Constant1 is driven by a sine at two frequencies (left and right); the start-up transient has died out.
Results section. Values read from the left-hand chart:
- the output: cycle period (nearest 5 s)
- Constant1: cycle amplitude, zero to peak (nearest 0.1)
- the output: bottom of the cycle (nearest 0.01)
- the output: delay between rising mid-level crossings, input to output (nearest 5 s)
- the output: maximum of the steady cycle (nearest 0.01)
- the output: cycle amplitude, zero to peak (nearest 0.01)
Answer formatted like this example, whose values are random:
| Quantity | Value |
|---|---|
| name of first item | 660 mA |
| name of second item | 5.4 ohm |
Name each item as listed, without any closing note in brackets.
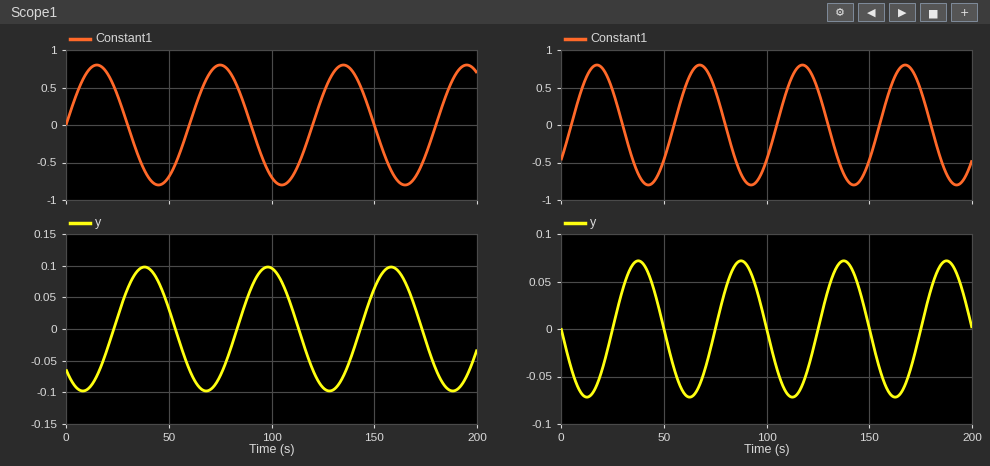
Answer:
| Quantity | Value |
|---|---|
| the output: cycle period | 60 s |
| Constant1: cycle amplitude, zero to peak | 0.8 |
| the output: bottom of the cycle | -0.10 |
| the output: delay between rising mid-level crossings, input to output | 25 s |
| the output: maximum of the steady cycle | 0.10 |
| the output: cycle amplitude, zero to peak | 0.10 |
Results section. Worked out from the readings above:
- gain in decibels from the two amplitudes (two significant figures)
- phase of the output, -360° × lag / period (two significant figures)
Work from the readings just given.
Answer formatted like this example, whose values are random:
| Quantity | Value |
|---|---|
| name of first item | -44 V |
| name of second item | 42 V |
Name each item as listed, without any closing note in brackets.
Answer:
| Quantity | Value |
|---|---|
| gain in decibels from the two amplitudes | -18 dB |
| phase of the output, -360° × lag / period | -150° |
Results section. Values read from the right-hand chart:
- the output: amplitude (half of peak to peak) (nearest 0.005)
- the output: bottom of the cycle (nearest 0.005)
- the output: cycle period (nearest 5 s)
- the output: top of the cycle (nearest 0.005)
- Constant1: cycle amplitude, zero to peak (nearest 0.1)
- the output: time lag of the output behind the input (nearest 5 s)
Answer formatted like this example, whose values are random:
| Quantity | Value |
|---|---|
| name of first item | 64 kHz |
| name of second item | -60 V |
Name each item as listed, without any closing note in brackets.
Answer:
| Quantity | Value |
|---|---|
| the output: amplitude (half of peak to peak) | 0.070 |
| the output: bottom of the cycle | -0.070 |
| the output: cycle period | 50 s |
| the output: top of the cycle | 0.070 |
| Constant1: cycle amplitude, zero to peak | 0.8 |
| the output: time lag of the output behind the input | 20 s |
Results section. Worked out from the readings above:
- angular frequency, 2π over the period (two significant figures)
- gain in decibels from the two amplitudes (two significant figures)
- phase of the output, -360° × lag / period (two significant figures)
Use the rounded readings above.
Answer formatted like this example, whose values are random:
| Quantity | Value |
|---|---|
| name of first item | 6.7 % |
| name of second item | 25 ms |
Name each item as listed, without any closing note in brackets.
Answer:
| Quantity | Value |
|---|---|
| angular frequency, 2π over the period | 0.13 rad/s |
| gain in decibels from the two amplitudes | -21 dB |
| phase of the output, -360° × lag / period | -140° |
